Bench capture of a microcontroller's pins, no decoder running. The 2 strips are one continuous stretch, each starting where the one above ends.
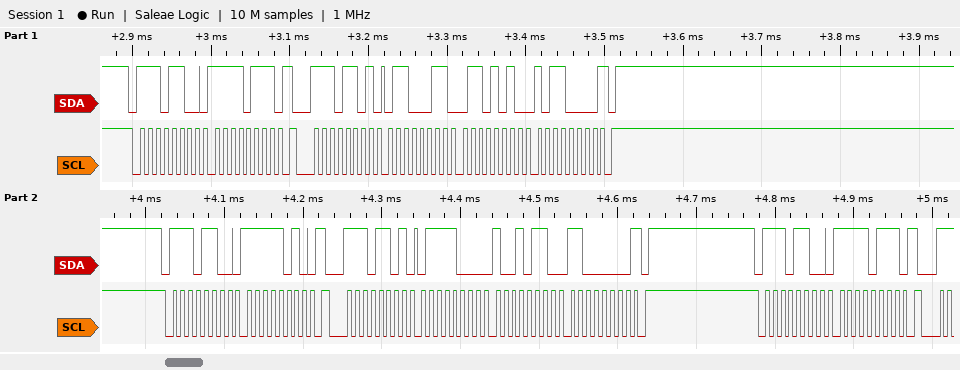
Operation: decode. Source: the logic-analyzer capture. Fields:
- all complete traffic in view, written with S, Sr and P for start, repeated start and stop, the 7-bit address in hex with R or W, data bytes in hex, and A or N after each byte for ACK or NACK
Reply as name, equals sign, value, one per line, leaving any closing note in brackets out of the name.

all complete traffic in view, written with S, Sr and P for start, repeated start and stop, the 7-bit address in hex with R or W, data bytes in hex, and A or N after each byte for ACK or NACK = S 76W A F7 A Sr 76R A 63 A 6A A B0 N P S 76W A FA A Sr 76R A 78 A 96 A C0 N P S 76W A F7 A
